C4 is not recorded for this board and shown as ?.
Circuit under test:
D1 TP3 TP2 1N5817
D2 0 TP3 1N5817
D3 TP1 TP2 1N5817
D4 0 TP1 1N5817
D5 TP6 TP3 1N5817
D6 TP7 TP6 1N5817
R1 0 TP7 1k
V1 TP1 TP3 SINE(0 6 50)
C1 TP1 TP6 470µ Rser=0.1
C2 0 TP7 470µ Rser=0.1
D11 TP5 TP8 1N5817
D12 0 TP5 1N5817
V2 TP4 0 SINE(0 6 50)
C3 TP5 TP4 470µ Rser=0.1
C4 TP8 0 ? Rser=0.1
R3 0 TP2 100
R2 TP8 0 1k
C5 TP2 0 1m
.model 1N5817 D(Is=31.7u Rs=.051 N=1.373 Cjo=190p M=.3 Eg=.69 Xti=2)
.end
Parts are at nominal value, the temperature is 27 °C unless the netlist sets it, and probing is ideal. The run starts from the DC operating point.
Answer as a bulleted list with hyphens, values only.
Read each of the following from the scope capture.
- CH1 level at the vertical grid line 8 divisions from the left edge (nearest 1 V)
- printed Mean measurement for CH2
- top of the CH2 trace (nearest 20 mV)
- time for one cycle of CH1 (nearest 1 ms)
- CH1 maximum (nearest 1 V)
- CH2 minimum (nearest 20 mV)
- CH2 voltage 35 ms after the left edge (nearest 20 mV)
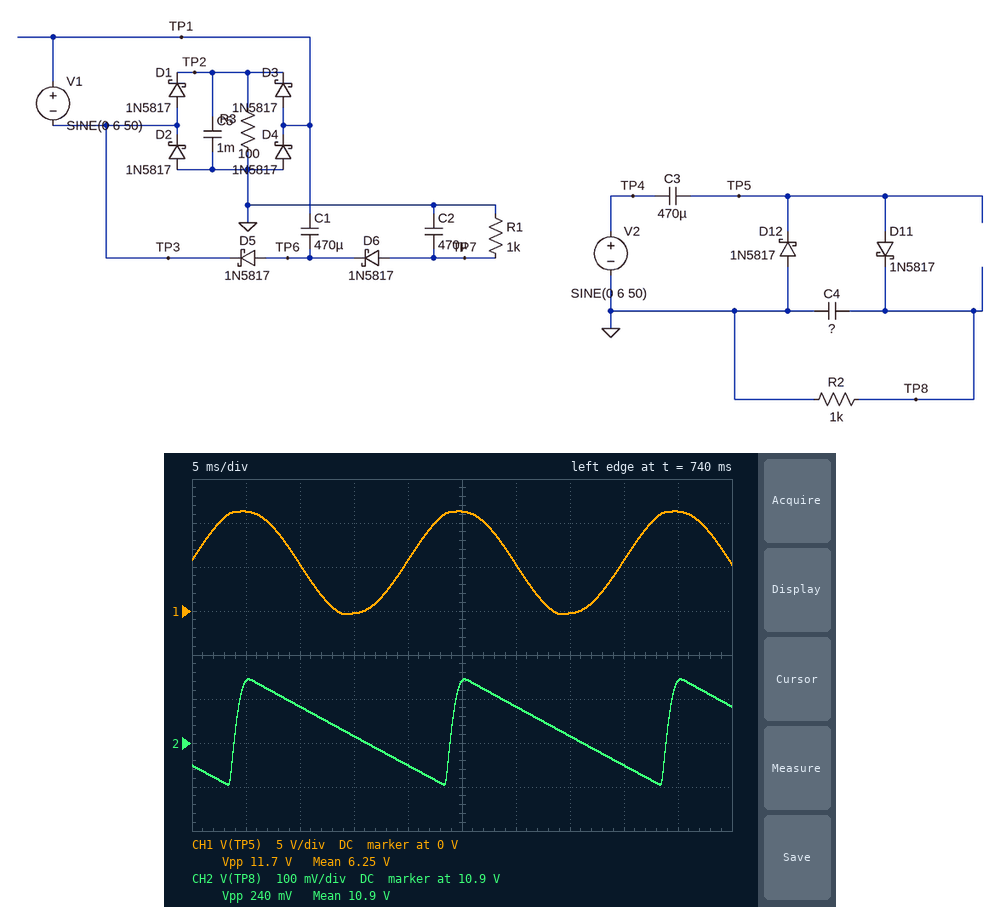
- 6 V
- 10.9 V
- 11.04 V
- 20 ms
- 11 V
- 10.80 V
- 10.92 V
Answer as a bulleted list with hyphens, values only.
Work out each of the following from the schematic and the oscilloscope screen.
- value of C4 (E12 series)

- 820 µF
